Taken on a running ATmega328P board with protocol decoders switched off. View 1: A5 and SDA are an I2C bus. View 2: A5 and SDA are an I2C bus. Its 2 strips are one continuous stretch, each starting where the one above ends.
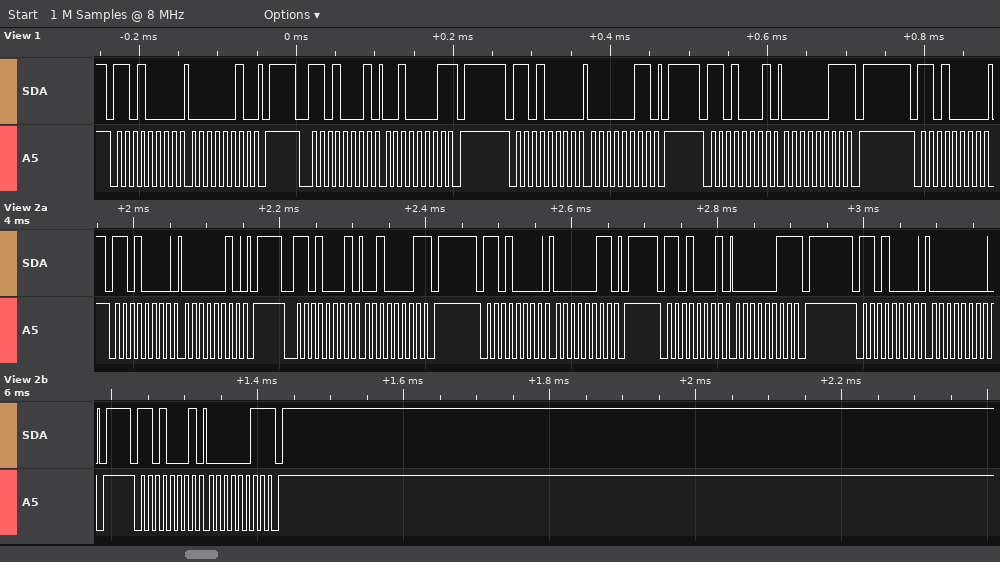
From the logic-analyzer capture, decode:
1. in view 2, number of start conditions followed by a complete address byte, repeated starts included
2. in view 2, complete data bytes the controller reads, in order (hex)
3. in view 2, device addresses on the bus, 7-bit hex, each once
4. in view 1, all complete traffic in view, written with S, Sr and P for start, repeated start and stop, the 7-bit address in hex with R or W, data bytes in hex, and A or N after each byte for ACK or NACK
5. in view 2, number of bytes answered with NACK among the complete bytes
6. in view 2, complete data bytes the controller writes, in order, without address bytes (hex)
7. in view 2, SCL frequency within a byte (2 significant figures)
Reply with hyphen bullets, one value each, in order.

- 6
- 21 03 03
- 0x68
- S 68W A 02 A P S 68R A 21 N P S 68W A 03 A P S 68R A 03 N P S 68W A
- 3
- 02 03 00
- 100 kHz
